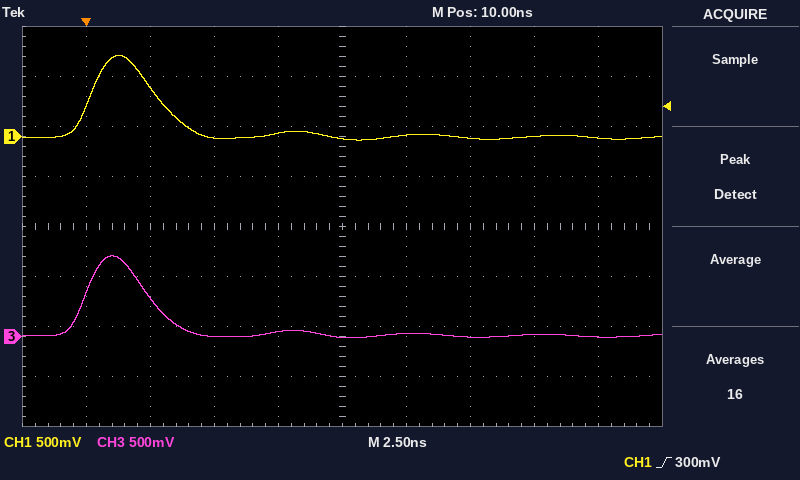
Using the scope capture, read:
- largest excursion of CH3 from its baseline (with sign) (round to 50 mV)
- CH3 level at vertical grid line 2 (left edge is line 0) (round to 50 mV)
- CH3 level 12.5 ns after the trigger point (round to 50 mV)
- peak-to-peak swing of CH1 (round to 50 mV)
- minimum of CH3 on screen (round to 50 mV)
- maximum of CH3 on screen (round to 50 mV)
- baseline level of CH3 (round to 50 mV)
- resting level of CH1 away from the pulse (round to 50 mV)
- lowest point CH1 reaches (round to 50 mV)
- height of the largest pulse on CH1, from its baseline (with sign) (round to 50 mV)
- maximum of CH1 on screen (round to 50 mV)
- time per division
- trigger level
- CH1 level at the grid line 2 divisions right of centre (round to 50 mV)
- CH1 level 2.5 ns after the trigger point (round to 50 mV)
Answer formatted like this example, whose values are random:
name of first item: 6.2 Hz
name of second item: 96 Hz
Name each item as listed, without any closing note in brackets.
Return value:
largest excursion of CH3 from its baseline (with sign): +800 mV
CH3 level at vertical grid line 2 (left edge is line 0): 400 mV
CH3 level 12.5 ns after the trigger point: 50 mV
peak-to-peak swing of CH1: 850 mV
minimum of CH3 on screen: 0 mV
maximum of CH3 on screen: 800 mV
baseline level of CH3: 0 mV
resting level of CH1 away from the pulse: 0 mV
lowest point CH1 reaches: -50 mV
height of the largest pulse on CH1, from its baseline (with sign): +800 mV
maximum of CH1 on screen: 800 mV
time per division: 2.5 ns
trigger level: 300 mV
CH1 level at the grid line 2 divisions right of centre: 0 mV
CH1 level 2.5 ns after the trigger point: 500 mV
